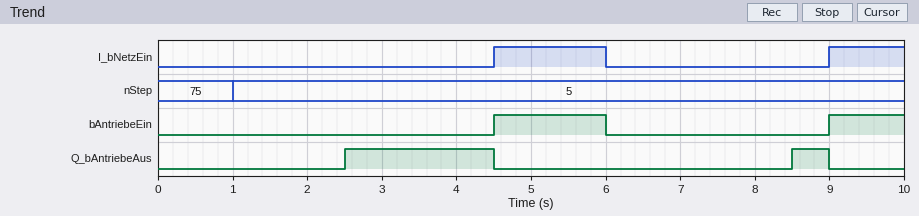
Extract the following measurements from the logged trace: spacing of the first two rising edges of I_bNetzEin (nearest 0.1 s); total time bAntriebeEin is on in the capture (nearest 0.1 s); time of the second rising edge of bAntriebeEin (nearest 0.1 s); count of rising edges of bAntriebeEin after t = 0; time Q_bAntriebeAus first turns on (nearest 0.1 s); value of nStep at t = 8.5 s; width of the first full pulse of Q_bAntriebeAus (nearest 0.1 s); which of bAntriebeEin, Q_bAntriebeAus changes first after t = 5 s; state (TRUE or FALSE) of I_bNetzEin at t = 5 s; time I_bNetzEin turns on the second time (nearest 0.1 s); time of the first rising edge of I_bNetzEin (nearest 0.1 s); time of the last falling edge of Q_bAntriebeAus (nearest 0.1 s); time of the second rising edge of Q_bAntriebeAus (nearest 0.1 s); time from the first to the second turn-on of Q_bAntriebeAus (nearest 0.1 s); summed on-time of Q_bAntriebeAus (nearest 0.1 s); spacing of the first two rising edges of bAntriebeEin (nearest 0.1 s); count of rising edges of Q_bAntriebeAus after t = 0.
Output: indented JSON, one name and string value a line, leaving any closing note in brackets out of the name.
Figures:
{
  "spacing of the first two rising edges of I_bNetzEin": "4.5 s",
  "total time bAntriebeEin is on in the capture": "2.5 s",
  "time of the second rising edge of bAntriebeEin": "9.0 s",
  "count of rising edges of bAntriebeEin after t = 0": "2",
  "time Q_bAntriebeAus first turns on": "2.5 s",
  "value of nStep at t = 8.5 s": "5",
  "width of the first full pulse of Q_bAntriebeAus": "2.0 s",
  "which of bAntriebeEin, Q_bAntriebeAus changes first after t = 5 s": "bAntriebeEin",
  "state (TRUE or FALSE) of I_bNetzEin at t = 5 s": "TRUE",
  "time I_bNetzEin turns on the second time": "9.0 s",
  "time of the first rising edge of I_bNetzEin": "4.5 s",
  "time of the last falling edge of Q_bAntriebeAus": "9.0 s",
  "time of the second rising edge of Q_bAntriebeAus": "8.5 s",
  "time from the first to the second turn-on of Q_bAntriebeAus": "6.0 s",
  "summed on-time of Q_bAntriebeAus": "2.5 s",
  "spacing of the first two rising edges of bAntriebeEin": "4.5 s",
  "count of rising edges of Q_bAntriebeAus after t = 0": "2"
}
